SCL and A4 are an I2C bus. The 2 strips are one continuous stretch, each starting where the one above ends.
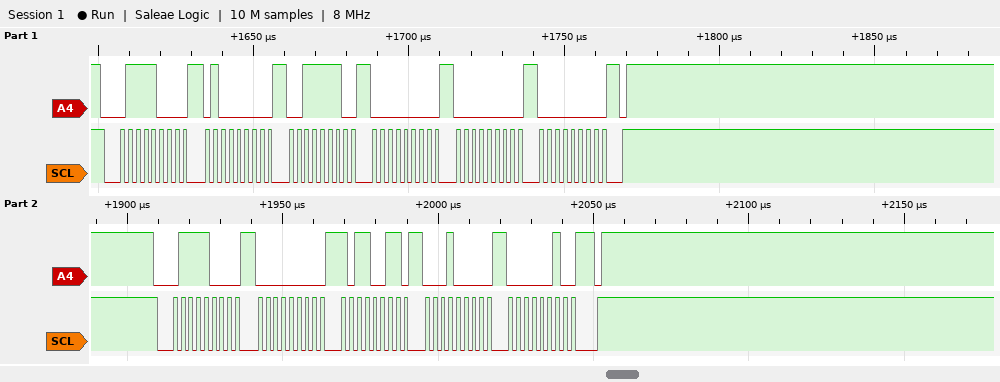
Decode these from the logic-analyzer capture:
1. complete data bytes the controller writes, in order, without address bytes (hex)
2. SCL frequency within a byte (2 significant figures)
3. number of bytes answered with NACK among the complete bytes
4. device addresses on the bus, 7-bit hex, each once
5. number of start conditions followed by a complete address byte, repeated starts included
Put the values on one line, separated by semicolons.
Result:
40 3E 00 00 00 00 B3 10 02; 400 kHz; 0; 0x3C; 2
